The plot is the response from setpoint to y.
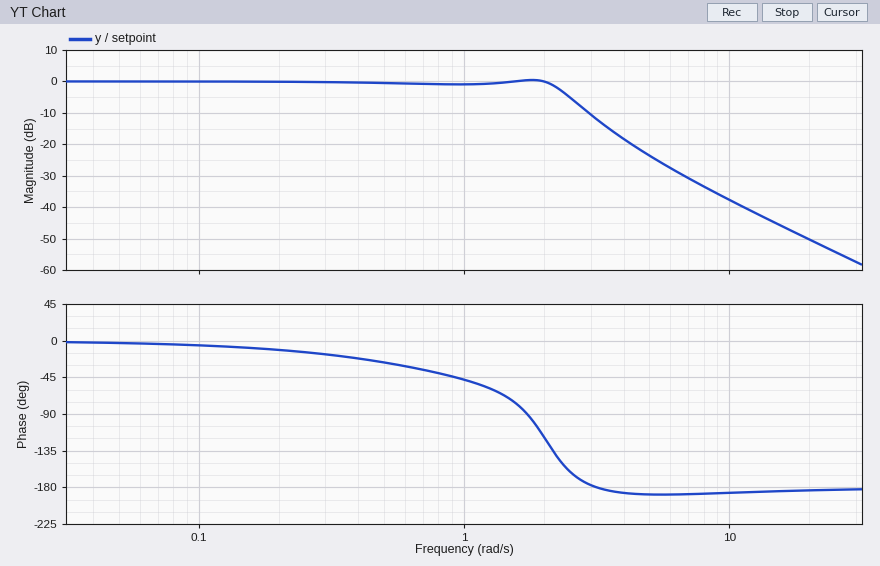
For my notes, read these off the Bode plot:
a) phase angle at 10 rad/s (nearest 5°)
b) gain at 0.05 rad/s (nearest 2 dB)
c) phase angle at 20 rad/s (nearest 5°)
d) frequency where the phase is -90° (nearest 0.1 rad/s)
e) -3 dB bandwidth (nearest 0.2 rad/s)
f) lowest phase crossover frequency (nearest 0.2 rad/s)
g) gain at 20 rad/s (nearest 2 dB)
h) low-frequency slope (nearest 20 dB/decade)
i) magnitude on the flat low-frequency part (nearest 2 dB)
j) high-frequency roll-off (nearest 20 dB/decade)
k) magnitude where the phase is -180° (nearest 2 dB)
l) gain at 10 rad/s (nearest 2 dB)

-185°
0 dB
-185°
1.7 rad/s
2.4 rad/s
3.2 rad/s
-50 dB
0 dB/decade
0 dB
-40 dB/decade
-12 dB
-38 dB
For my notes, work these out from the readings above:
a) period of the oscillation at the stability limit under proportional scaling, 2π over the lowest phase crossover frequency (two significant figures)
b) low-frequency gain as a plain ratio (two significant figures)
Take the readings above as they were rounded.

2.0 s
1.0
